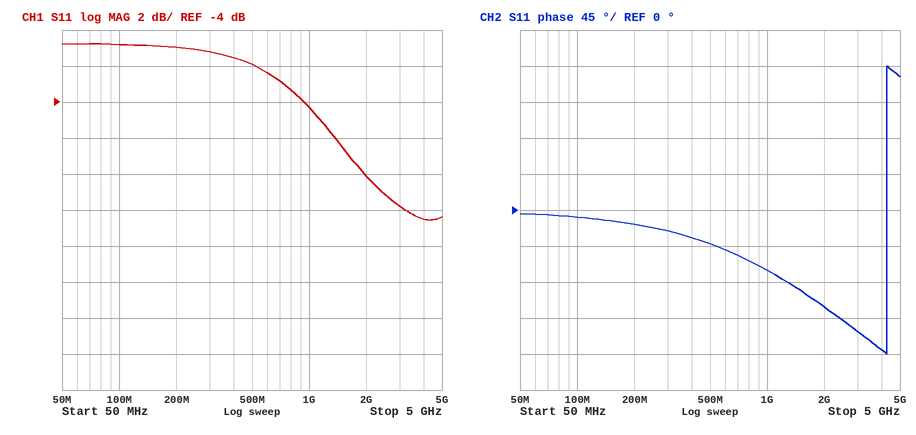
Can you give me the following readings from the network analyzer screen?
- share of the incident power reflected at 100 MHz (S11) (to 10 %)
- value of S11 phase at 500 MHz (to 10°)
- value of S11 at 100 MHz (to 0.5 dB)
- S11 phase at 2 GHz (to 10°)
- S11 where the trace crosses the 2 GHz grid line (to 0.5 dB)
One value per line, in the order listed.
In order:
80 %
-40°
-1.0 dB
-120°
-8.0 dB
